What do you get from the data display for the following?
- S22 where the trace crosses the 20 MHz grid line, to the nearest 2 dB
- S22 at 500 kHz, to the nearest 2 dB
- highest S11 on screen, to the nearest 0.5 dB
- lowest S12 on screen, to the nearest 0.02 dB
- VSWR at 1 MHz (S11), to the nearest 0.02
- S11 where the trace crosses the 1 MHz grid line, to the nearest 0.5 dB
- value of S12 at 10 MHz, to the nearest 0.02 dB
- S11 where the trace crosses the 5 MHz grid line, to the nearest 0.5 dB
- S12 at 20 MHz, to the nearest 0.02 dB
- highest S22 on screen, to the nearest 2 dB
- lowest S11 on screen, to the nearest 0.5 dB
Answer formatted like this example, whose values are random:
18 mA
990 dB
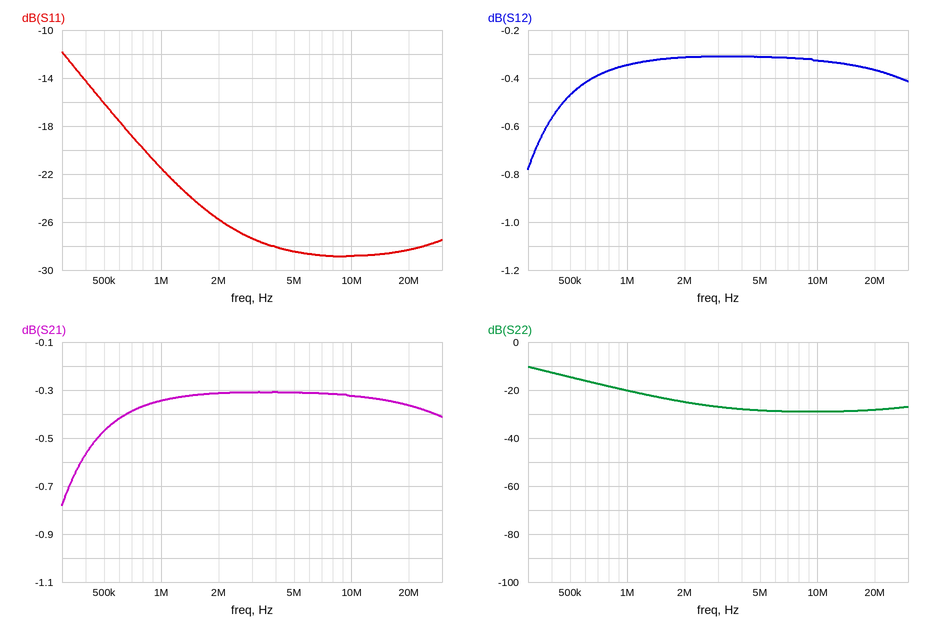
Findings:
-28 dB
-14 dB
-12.0 dB
-0.78 dB
1.18
-21.5 dB
-0.32 dB
-28.5 dB
-0.36 dB
-10 dB
-29.0 dB
